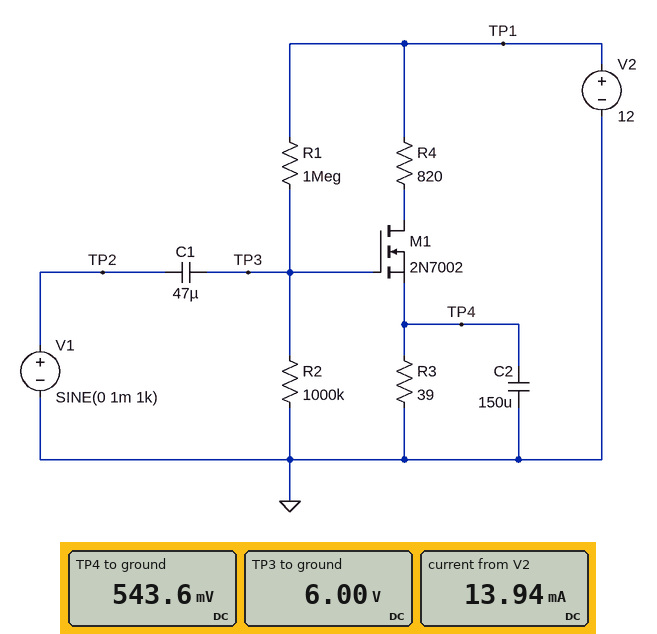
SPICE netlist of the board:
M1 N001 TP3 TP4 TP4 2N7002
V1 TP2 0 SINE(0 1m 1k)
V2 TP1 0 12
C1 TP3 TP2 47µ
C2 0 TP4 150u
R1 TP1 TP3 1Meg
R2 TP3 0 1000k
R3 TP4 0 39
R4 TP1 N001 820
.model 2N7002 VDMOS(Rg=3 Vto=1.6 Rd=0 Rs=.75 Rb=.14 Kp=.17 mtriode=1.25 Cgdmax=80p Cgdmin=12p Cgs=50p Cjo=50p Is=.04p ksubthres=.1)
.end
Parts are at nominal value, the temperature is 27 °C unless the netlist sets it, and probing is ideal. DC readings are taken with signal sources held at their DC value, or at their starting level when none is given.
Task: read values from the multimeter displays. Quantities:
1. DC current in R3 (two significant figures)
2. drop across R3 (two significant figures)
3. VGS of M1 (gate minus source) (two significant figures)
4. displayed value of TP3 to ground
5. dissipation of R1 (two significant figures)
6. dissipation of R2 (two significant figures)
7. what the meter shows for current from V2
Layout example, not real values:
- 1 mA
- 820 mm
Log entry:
- 14 mA
- 540 mV
- 5.5 V
- 6.00 V
- 36 µW
- 36 µW
- 13.94 mA
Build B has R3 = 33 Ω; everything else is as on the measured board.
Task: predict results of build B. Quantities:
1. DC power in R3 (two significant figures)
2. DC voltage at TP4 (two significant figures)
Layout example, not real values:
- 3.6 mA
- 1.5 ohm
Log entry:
- 6.5 mW
- 460 mV
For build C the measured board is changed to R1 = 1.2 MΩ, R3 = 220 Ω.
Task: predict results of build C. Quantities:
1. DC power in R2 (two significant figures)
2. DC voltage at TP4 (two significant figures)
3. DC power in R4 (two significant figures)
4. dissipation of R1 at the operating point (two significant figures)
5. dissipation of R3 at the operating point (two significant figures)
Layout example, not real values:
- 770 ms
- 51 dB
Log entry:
- 30 µW
- 2.5 V
- 110 mW
- 36 µW
- 29 mW
